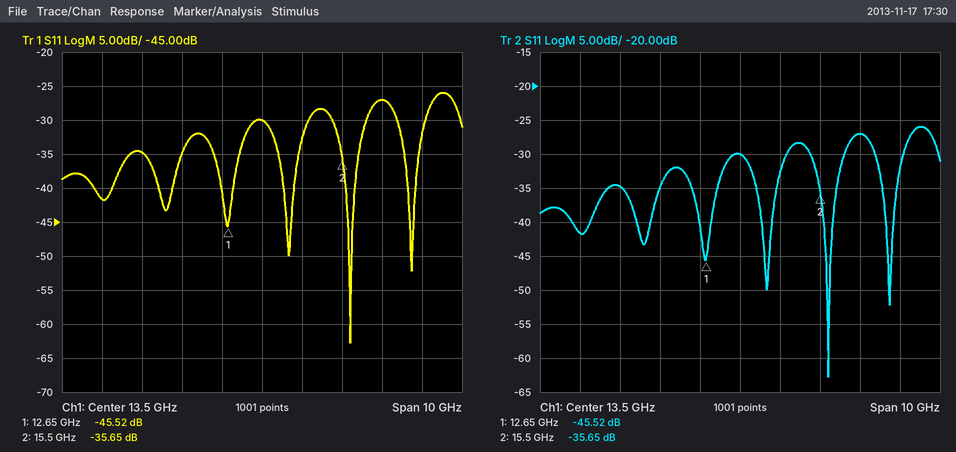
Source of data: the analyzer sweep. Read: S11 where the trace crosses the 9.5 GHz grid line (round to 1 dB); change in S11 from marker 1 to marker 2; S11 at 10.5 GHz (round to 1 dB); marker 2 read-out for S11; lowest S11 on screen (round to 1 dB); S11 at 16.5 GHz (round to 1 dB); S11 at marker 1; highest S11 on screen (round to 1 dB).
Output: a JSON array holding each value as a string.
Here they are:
["-42 dB", "9.87 dB", "-35 dB", "-35.65 dB", "-63 dB", "-27 dB", "-45.52 dB", "-26 dB"]
